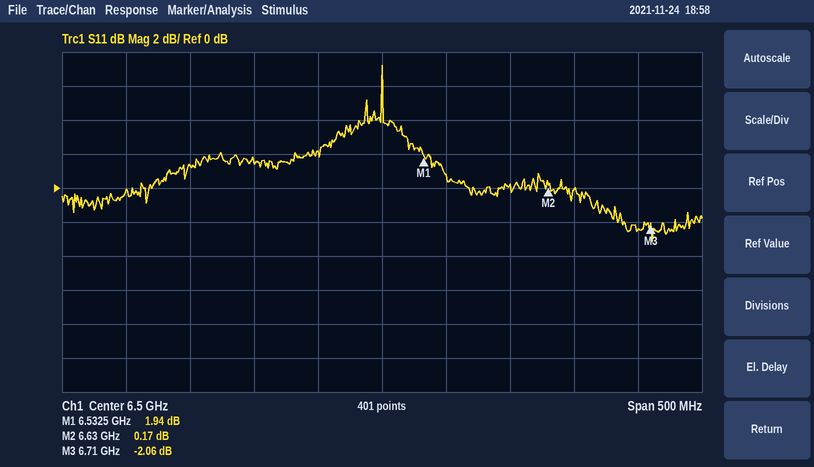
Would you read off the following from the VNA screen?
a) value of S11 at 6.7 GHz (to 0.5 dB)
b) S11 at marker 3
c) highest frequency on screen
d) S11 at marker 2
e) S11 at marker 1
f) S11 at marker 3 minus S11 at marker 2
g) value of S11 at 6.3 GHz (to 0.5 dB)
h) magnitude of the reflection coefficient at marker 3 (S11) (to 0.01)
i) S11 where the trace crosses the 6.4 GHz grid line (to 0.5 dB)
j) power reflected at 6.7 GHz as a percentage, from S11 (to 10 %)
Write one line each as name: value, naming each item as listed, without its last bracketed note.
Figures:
value of S11 at 6.7 GHz: -2.5 dB
S11 at marker 3: -2.06 dB
highest frequency on screen: 6.75 GHz
S11 at marker 2: 0.17 dB
S11 at marker 1: 1.94 dB
S11 at marker 3 minus S11 at marker 2: -2.23 dB
value of S11 at 6.3 GHz: 0.0 dB
magnitude of the reflection coefficient at marker 3 (S11): 0.79
S11 where the trace crosses the 6.4 GHz grid line: 1.5 dB
power reflected at 6.7 GHz as a percentage, from S11: 60 %
